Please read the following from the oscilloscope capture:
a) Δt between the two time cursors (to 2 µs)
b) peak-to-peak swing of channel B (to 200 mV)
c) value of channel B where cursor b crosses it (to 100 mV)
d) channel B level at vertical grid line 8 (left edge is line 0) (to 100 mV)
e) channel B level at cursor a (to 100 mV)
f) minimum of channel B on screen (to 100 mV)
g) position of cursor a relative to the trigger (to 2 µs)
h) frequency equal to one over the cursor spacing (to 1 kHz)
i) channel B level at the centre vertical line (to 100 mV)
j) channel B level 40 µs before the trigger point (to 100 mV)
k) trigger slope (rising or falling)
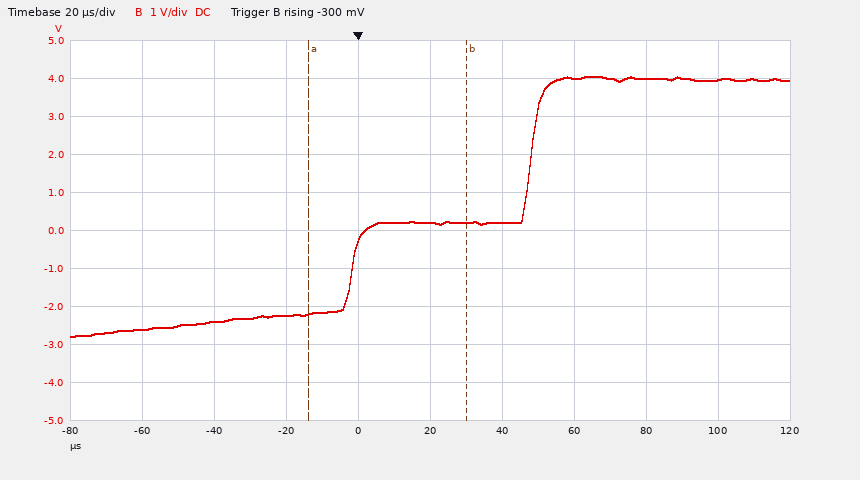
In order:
44 µs
6.8 V
200 mV
4.0 V
-2.2 V
-2.8 V
-14 µs
23 kHz
200 mV
-2.4 V
rising
